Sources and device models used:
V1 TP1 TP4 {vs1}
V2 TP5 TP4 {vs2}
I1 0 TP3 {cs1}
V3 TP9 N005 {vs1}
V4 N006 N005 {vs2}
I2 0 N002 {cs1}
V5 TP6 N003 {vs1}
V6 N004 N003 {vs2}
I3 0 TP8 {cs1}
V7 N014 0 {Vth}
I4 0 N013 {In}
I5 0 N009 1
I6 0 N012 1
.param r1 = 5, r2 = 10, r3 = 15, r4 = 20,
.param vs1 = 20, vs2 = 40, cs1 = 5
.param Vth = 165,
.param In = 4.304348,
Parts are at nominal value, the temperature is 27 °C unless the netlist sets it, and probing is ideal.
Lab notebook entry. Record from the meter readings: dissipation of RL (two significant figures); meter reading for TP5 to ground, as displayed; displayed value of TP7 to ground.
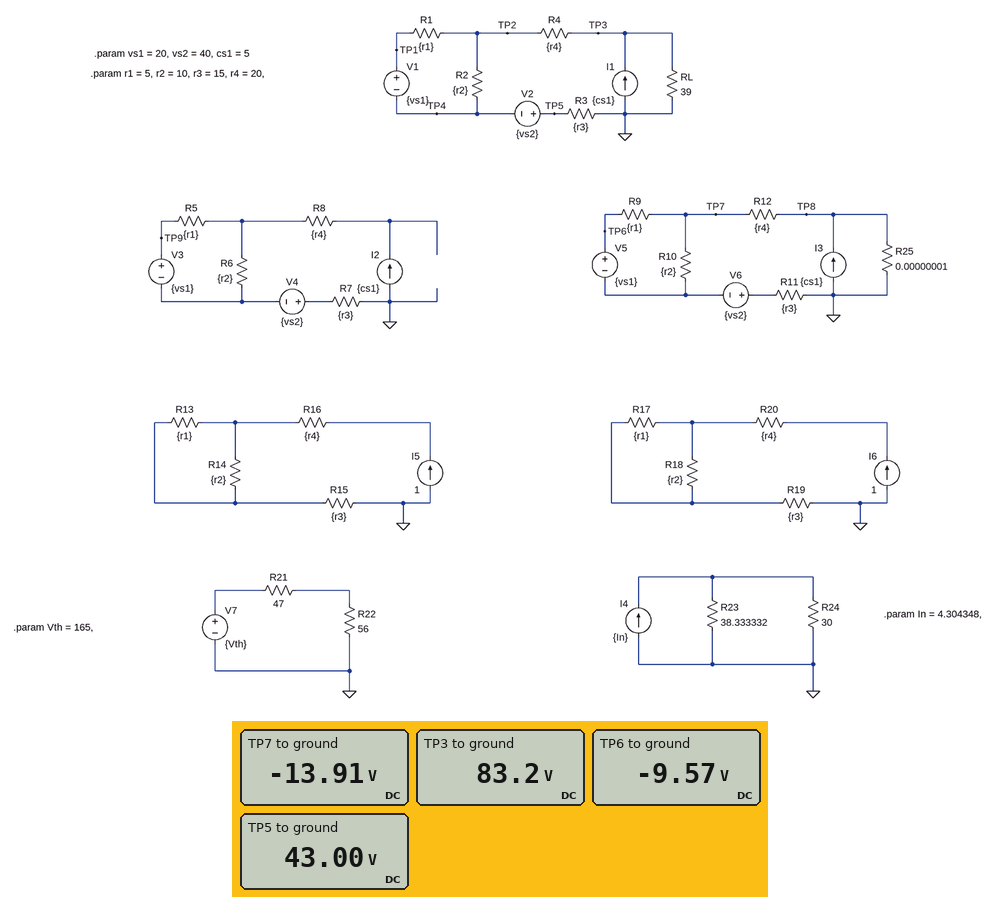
180 W
43.00 V
-13.91 V
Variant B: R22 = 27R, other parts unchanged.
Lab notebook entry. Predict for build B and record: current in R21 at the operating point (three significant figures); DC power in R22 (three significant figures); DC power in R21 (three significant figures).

2.23 A
134 W
234 W
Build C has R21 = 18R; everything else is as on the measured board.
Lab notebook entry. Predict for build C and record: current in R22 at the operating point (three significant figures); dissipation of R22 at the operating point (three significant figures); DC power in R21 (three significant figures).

2.23 A
278 W
89.5 W
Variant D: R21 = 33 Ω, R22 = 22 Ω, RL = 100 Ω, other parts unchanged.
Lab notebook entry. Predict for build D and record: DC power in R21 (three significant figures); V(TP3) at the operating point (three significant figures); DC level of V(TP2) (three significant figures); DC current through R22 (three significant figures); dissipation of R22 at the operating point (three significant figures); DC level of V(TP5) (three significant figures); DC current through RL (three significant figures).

297 W
119 V
43.1 V
3.00 A
198 W
57.1 V
1.19 A
